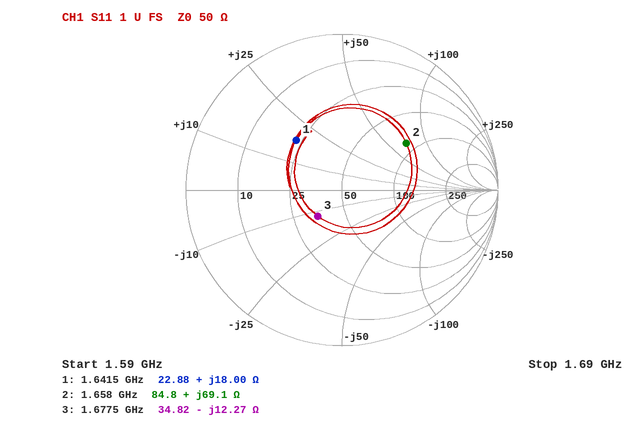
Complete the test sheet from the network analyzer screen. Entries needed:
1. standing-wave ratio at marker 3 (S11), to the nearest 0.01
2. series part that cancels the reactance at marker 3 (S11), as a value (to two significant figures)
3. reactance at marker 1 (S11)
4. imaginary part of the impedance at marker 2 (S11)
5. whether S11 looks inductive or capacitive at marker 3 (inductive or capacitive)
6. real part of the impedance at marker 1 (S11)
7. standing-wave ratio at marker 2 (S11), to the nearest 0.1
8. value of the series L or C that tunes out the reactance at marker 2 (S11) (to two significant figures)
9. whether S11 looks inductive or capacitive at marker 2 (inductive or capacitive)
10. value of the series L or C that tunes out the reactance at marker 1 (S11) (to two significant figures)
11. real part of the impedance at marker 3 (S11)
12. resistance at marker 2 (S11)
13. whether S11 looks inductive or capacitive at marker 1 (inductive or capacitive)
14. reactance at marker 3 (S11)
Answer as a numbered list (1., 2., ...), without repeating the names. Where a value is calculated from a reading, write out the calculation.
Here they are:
1. 1.59
2. L = 12.27 Ω/(2π × 1.6775 GHz) ≈ 1.2 nH
3. +18.00 Ω
4. +69.1 Ω
5. capacitive
6. 22.88 Ω
7. 3.1
8. C = 1/(2π × 1.658 GHz × 69.1 Ω) ≈ 1.4 pF
9. inductive
10. C = 1/(2π × 1.6415 GHz × 18 Ω) ≈ 5.4 pF
11. 34.82 Ω
12. 84.8 Ω
13. inductive
14. -12.27 Ω
